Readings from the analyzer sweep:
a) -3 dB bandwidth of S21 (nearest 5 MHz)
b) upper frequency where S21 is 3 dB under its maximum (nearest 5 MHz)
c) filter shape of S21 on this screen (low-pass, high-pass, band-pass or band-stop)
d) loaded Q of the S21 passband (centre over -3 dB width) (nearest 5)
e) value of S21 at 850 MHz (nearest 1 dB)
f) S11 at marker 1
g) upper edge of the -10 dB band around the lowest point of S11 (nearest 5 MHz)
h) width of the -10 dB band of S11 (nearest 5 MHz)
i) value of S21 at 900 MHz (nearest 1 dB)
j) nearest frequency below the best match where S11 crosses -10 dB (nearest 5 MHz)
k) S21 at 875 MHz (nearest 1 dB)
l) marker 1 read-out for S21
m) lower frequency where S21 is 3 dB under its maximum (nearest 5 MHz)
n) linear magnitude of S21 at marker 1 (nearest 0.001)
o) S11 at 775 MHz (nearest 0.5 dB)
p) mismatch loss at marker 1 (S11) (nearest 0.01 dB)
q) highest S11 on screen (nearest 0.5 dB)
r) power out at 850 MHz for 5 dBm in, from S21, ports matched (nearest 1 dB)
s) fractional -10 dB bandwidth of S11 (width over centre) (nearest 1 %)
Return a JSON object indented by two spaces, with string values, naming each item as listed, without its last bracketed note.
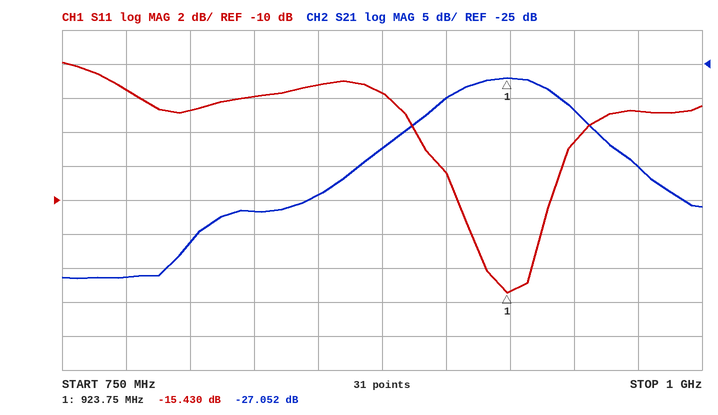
{
  "-3 dB bandwidth of S21": "45 MHz",
  "upper frequency where S21 is 3 dB under its maximum": "945 MHz",
  "filter shape of S21 on this screen": "band-pass",
  "loaded Q of the S21 passband (centre over -3 dB width)": "20",
  "value of S21 at 850 MHz": "-44 dB",
  "S11 at marker 1": "-15.430 dB",
  "upper edge of the -10 dB band around the lowest point of S11": "940 MHz",
  "width of the -10 dB band of S11": "35 MHz",
  "value of S21 at 900 MHz": "-30 dB",
  "nearest frequency below the best match where S11 crosses -10 dB": "905 MHz",
  "S21 at 875 MHz": "-37 dB",
  "marker 1 read-out for S21": "-27.052 dB",
  "lower frequency where S21 is 3 dB under its maximum": "900 MHz",
  "linear magnitude of S21 at marker 1": "0.044",
  "S11 at 775 MHz": "-3.5 dB",
  "mismatch loss at marker 1 (S11)": "0.13 dB",
  "highest S11 on screen": "-2.0 dB",
  "power out at 850 MHz for 5 dBm in, from S21, ports matched": "-39 dBm",
  "fractional -10 dB bandwidth of S11 (width over centre)": "4 %"
}
